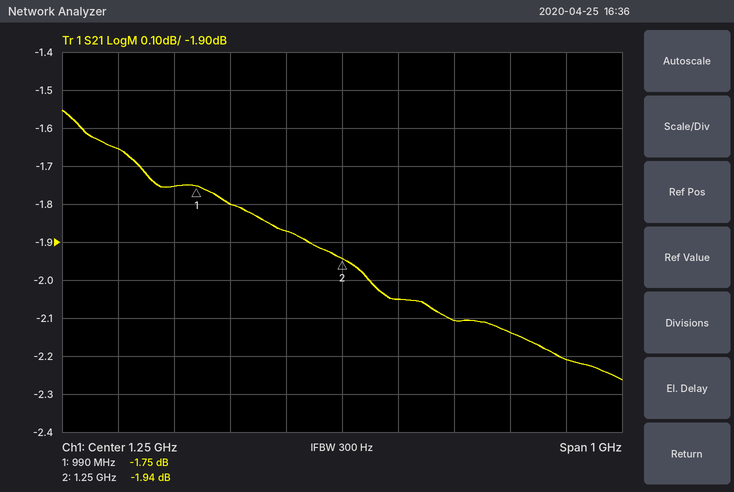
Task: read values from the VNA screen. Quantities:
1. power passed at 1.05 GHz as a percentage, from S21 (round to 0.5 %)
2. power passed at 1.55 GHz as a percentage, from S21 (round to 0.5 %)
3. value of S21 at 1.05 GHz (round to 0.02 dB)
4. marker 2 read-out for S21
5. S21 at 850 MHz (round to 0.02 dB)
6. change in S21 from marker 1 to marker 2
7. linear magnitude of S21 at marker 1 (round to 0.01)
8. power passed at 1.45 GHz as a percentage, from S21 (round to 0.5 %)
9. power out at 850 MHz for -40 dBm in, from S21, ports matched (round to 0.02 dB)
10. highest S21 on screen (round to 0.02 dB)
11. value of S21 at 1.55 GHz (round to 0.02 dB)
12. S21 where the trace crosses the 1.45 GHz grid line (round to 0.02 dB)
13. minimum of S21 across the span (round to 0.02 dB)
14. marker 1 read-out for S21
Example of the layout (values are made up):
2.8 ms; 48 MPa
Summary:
66.0 %; 61.0 %; -1.80 dB; -1.94 dB; -1.66 dB; -0.19 dB; 0.82; 61.5 %; -41.66 dBm; -1.56 dB; -2.14 dB; -2.10 dB; -2.26 dB; -1.75 dB
